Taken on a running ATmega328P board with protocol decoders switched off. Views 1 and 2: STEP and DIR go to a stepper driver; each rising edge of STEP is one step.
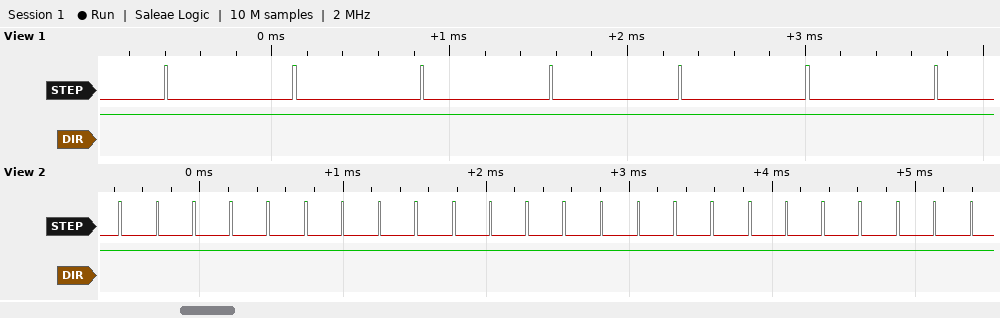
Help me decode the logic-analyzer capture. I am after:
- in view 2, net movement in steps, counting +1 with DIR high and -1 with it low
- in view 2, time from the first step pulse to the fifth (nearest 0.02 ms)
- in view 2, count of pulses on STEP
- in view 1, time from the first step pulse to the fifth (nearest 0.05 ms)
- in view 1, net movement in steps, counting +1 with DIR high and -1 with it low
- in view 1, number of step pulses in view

+24
1.04 ms
24
2.90 ms
+7
7
